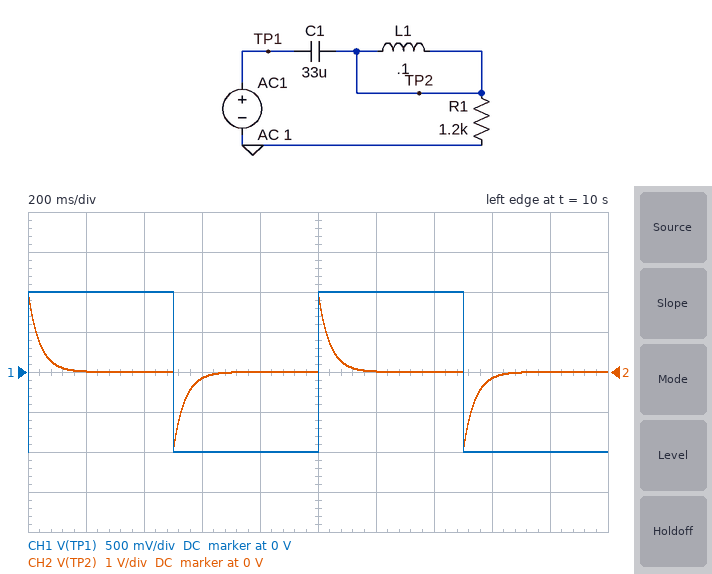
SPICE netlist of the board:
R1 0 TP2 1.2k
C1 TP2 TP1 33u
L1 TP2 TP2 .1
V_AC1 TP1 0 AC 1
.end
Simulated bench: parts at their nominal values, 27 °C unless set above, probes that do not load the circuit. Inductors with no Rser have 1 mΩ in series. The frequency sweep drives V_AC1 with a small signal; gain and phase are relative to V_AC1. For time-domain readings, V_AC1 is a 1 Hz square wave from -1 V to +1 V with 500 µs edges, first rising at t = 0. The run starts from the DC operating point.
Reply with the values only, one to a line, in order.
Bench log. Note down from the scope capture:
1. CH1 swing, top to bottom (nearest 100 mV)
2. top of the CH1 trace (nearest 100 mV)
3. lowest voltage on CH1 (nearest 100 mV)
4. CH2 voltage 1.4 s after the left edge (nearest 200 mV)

2.0 V
1.0 V
-1.0 V
0 V
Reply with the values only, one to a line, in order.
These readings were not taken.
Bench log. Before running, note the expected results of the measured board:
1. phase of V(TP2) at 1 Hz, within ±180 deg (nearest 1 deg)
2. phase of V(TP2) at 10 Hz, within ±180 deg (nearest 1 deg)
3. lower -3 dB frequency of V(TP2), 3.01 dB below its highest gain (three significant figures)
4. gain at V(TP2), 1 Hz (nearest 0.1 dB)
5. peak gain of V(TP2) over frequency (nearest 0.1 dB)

76 deg
22 deg
4.02 Hz
-12.3 dB
0 dB
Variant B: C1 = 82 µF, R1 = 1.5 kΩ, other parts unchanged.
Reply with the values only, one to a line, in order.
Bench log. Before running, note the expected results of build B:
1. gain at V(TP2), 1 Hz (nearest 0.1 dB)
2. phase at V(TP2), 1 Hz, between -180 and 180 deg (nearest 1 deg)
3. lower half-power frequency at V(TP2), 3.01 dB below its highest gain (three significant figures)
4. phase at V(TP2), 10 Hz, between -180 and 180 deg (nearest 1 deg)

-4.3 dB
52 deg
1.29 Hz
7 deg
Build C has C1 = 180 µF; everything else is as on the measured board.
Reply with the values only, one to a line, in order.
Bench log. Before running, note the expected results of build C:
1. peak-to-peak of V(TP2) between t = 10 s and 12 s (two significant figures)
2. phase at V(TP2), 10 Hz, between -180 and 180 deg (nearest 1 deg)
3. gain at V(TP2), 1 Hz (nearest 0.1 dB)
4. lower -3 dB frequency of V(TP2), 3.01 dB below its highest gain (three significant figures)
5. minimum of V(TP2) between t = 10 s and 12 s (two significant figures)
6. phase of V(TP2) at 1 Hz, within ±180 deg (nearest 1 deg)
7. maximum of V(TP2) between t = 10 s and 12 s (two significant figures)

3.6 V
4 deg
-1.9 dB
737 mHz
-1.8 V
36 deg
1.8 V
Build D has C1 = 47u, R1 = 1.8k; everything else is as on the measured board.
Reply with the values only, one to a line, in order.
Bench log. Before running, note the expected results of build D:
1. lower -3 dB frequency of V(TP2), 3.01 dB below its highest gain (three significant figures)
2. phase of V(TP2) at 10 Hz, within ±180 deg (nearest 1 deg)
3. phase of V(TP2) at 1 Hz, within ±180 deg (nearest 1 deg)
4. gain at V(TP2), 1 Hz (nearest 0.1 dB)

1.88 Hz
11 deg
62 deg
-6.6 dB
